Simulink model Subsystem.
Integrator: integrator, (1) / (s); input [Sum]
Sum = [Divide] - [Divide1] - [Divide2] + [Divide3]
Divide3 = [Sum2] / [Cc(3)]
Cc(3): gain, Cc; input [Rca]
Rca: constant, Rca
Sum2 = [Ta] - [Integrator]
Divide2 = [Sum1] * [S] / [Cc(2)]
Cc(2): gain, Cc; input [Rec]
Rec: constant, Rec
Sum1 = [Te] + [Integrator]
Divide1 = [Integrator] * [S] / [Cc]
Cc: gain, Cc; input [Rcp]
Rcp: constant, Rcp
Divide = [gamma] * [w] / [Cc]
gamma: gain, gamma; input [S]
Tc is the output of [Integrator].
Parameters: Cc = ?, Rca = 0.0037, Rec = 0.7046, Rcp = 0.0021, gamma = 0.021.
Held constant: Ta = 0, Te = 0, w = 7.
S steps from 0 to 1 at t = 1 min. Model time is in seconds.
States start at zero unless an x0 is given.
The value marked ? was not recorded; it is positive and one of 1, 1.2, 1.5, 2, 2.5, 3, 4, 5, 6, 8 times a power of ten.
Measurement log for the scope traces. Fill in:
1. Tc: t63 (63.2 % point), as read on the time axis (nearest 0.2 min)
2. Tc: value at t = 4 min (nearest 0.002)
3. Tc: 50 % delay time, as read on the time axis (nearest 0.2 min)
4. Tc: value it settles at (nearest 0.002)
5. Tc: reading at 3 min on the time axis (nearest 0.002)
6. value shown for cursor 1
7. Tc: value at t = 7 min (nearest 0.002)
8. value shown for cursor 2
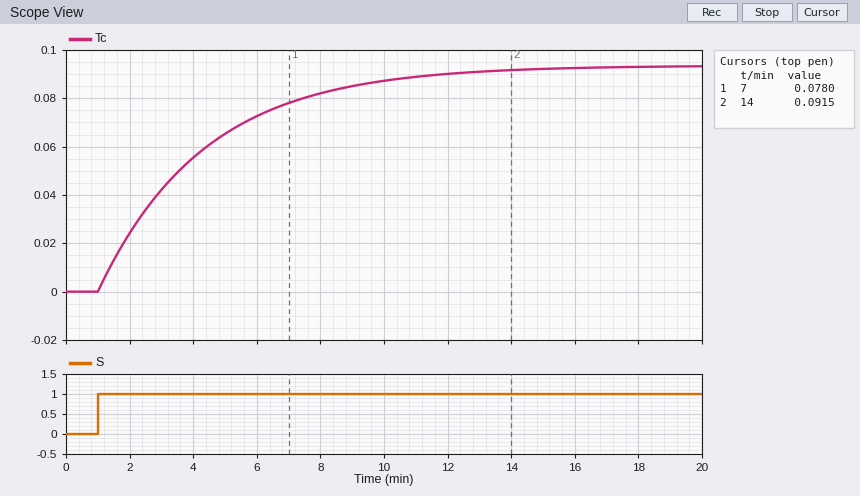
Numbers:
4.4 min
0.056
3.4 min
0.094
0.042
0.0780
0.078
0.0915
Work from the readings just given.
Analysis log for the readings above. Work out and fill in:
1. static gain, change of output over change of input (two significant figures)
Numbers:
0.094
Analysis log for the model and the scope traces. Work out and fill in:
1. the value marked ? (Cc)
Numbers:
150000
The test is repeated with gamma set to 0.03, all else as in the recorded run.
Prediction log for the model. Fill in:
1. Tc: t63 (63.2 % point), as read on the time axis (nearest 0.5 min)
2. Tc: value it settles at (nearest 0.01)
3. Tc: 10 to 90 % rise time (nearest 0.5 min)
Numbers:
4.5 min
0.13
7.5 min
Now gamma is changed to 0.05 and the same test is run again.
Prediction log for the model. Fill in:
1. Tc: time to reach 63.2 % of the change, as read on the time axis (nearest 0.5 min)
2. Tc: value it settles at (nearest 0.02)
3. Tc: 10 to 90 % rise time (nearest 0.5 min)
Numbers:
4.5 min
0.22
7.5 min
